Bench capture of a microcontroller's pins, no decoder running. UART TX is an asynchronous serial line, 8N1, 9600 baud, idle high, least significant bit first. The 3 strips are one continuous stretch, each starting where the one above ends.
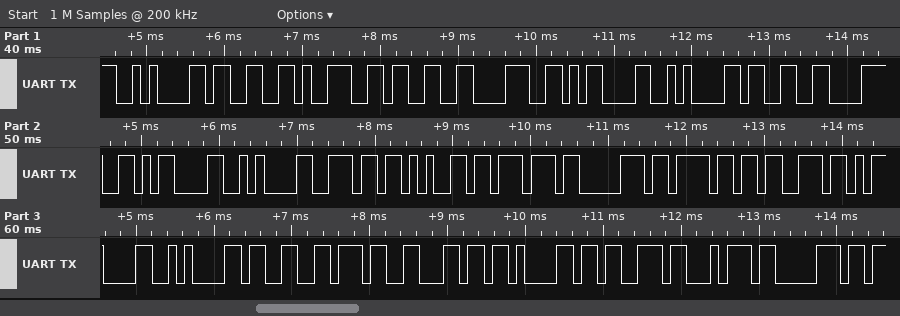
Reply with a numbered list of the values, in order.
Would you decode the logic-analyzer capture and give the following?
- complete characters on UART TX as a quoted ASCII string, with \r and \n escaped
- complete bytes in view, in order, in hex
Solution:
1. "\n3938\r\n38\r\nnewpos\r\n37lastp"
2. 0A 33 39 33 38 0D 0A 33 38 0D 0A 6E 65 77 70 6F 73 0D 0A 33 37 6C 61 73 74 70
